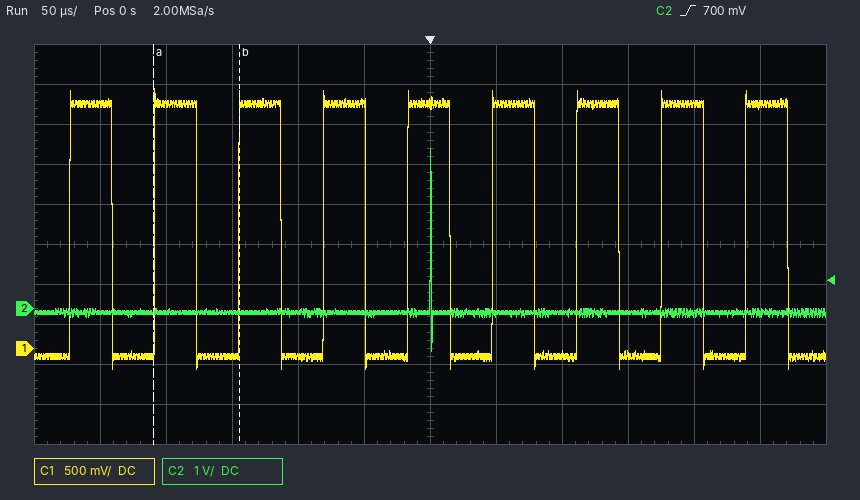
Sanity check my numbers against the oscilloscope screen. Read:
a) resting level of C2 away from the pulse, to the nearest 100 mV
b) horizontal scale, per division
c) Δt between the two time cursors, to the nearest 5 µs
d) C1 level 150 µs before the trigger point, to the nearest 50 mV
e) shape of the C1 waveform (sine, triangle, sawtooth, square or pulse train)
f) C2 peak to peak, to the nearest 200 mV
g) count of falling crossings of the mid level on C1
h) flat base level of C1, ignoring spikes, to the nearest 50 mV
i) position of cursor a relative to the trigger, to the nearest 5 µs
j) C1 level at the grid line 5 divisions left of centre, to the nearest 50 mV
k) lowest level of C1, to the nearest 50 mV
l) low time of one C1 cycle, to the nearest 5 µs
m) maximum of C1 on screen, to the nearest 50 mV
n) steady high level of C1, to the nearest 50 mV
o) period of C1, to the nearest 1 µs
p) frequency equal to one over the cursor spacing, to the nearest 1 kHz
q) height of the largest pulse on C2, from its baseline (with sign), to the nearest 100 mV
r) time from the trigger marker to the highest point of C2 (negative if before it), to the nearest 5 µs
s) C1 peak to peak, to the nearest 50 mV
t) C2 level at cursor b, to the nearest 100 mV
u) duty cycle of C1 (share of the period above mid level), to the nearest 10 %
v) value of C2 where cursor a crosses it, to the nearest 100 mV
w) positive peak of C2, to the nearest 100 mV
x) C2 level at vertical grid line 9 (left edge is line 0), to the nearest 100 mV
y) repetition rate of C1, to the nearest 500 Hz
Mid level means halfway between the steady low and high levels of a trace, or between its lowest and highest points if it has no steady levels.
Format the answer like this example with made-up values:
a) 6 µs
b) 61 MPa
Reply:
a) -100 mV
b) 50 µs
c) 65 µs
d) -100 mV
e) square
f) 5.0 V
g) 9
h) -100 mV
i) -210 µs
j) 3.05 V
k) -250 mV
l) 30 µs
m) 3.25 V
n) 3.05 V
o) 64 µs
p) 15 kHz
q) +4.1 V
r) 0 µs
s) 3.50 V
t) -100 mV
u) 50 %
v) -100 mV
w) 4.0 V
x) -100 mV
y) 15.5 kHz
